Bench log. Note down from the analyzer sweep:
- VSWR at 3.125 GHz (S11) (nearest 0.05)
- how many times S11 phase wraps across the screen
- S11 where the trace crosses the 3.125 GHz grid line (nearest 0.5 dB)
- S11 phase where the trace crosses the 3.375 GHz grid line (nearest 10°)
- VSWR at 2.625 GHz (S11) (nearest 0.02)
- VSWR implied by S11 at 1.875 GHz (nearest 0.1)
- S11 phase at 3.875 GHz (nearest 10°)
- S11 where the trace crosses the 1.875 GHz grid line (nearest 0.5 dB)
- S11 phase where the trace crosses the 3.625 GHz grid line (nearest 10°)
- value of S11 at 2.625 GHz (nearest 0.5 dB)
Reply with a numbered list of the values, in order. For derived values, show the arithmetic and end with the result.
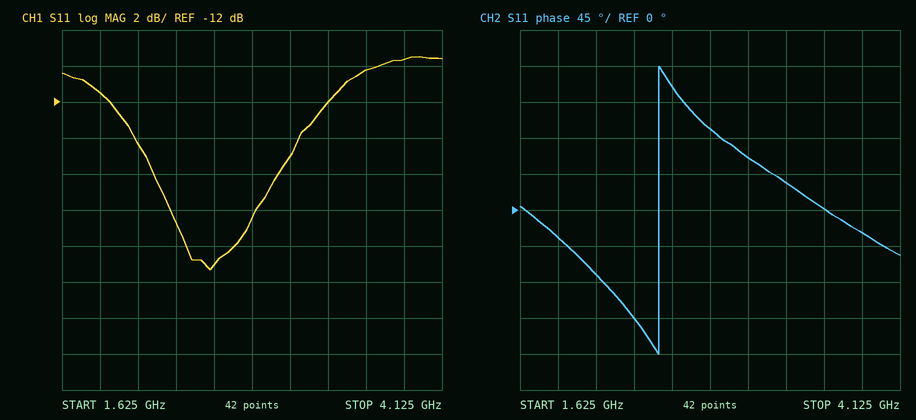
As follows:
1. |Γ| = 10^(-15/20) = 0.1778; VSWR = (1 + 0.1778)/(1 − 0.1778) ≈ 1.43, so 1.45 to the nearest 0.05
2. 1
3. -15.0 dB
4. 30°
5. |Γ| = 10^(-21/20) = 0.0891; VSWR = (1 + 0.0891)/(1 − 0.0891) ≈ 1.20
6. |Γ| = 10^(-11.5/20) = 0.2661; VSWR = (1 + 0.2661)/(1 − 0.2661) ≈ 1.7
7. -30°
8. -11.5 dB
9. 0°
10. -21.0 dB
